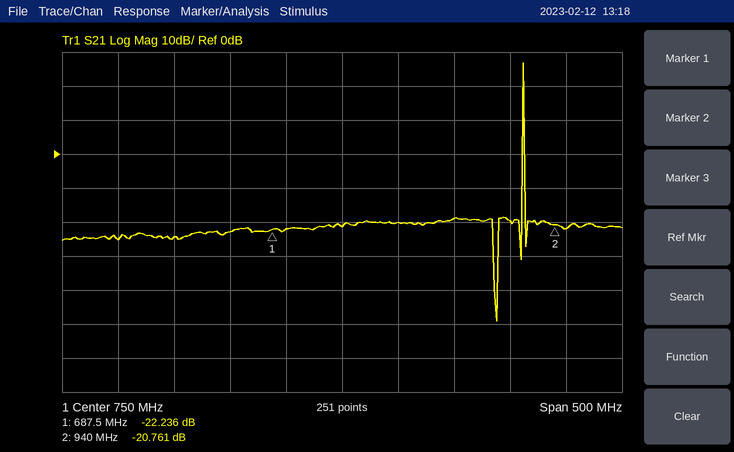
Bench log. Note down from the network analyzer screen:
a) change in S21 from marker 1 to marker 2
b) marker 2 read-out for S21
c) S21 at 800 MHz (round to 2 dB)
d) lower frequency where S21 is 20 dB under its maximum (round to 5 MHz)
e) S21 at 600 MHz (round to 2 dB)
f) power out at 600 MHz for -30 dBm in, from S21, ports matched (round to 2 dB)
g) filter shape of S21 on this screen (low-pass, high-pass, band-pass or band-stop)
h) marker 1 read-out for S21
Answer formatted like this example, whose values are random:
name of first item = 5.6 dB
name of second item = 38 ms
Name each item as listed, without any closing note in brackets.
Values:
change in S21 from marker 1 to marker 2 = 1.475 dB
marker 2 read-out for S21 = -20.761 dB
S21 at 800 MHz = -20 dB
lower frequency where S21 is 20 dB under its maximum = 910 MHz
S21 at 600 MHz = -24 dB
power out at 600 MHz for -30 dBm in, from S21, ports matched = -54 dBm
filter shape of S21 on this screen = band-pass
marker 1 read-out for S21 = -22.236 dB
